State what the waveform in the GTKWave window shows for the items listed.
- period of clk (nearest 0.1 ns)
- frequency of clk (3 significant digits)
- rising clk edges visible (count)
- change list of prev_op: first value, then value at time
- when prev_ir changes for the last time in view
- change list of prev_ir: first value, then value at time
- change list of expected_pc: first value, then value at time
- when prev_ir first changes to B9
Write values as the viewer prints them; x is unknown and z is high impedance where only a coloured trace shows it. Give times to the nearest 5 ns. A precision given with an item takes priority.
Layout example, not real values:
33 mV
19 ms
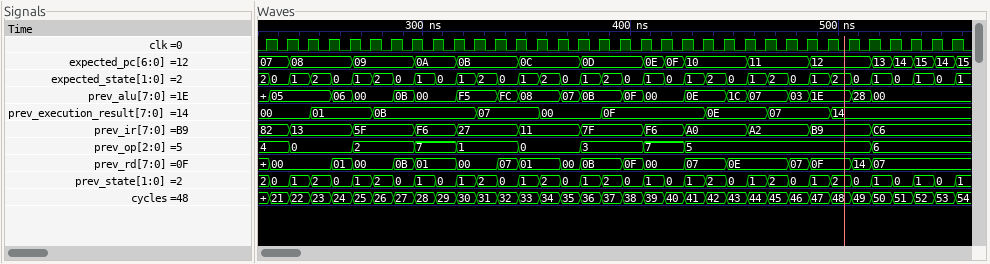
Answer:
10 ns
100 MHz
34
4, 0 at 235 ns, 2 at 265 ns, 7 at 295 ns, 1 at 315 ns, 0 at 345 ns, 3 at 375 ns, 7 at 405 ns, 5 at 425 ns, 6 at 515 ns
515 ns
82, 13 at 235 ns, 5F at 265 ns, F6 at 295 ns, 27 at 315 ns, 11 at 345 ns, 7F at 375 ns, F6 at 405 ns, A0 at 425 ns, A2 at 455 ns, B9 at 485 ns, C6 at 515 ns
07, 08 at 235 ns, 09 at 265 ns, 0A at 295 ns, 0B at 315 ns, 0C at 345 ns, 0D at 375 ns, 0E at 405 ns, 0F at 415 ns, 10 at 425 ns, 11 at 455 ns, 12 at 485 ns, 13 at 515 ns, 14 at 525 ns, 15 at 535 ns, 14 at 545 ns, 15 at 555 ns
485 ns
